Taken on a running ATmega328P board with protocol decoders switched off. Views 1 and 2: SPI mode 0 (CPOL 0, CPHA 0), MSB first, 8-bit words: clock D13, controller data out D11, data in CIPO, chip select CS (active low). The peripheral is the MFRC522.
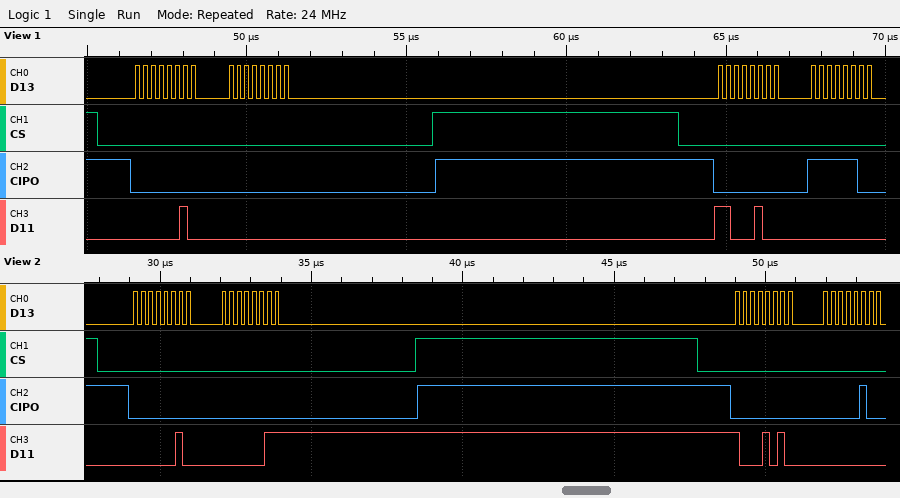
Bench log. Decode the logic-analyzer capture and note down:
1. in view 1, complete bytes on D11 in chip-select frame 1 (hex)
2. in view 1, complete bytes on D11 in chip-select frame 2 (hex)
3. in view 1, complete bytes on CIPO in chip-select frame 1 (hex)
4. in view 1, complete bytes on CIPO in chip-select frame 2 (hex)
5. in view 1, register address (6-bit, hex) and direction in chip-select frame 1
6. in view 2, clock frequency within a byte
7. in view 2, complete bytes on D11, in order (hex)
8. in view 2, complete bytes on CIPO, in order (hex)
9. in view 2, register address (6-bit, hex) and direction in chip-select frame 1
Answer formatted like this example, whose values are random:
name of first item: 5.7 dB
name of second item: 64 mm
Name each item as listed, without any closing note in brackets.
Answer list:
in view 1, complete bytes on D11 in chip-select frame 1: 02 00
in view 1, complete bytes on D11 in chip-select frame 2: C4 00
in view 1, complete bytes on CIPO in chip-select frame 1: 00 00
in view 1, complete bytes on CIPO in chip-select frame 2: 00 FC
in view 1, register address (6-bit, hex) and direction in chip-select frame 1: 0x01 write
in view 2, clock frequency within a byte: 4 MHz
in view 2, complete bytes on D11, in order: 02 03 8A 00
in view 2, complete bytes on CIPO, in order: 00 00 00 04
in view 2, register address (6-bit, hex) and direction in chip-select frame 1: 0x01 write
